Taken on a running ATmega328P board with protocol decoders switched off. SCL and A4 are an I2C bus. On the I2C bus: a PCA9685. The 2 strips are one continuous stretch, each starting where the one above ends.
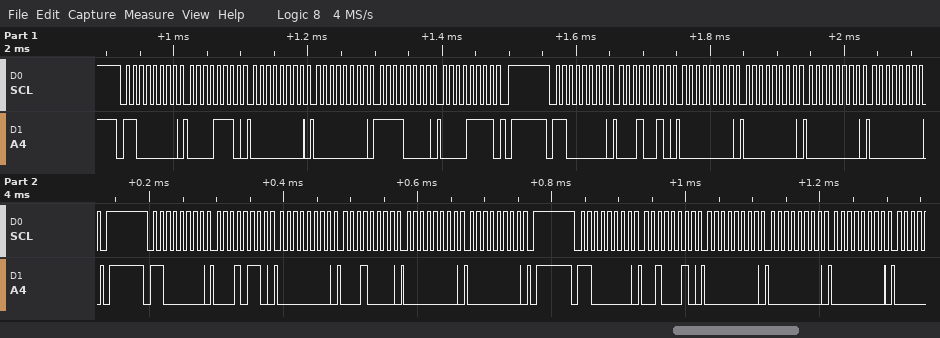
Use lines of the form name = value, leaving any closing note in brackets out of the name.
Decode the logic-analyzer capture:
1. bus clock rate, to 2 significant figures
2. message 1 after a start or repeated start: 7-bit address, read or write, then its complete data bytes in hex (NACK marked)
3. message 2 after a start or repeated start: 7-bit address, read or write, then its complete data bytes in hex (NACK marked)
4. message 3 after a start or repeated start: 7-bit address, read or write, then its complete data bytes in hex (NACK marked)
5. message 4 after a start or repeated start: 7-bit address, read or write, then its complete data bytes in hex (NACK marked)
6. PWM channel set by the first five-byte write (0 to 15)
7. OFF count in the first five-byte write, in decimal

bus clock rate, to 2 significant figures = 100 kHz
message 1 after a start or repeated start: 7-bit address, read or write, then its complete data bytes in hex = 0x60 write: 0E 00 00 F0 0F
message 2 after a start or repeated start: 7-bit address, read or write, then its complete data bytes in hex = 0x60 write: 12 00 00 00 00
message 3 after a start or repeated start: 7-bit address, read or write, then its complete data bytes in hex = 0x60 write: 16 00 10 00 00
message 4 after a start or repeated start: 7-bit address, read or write, then its complete data bytes in hex = 0x60 write: 22 00 00 00
PWM channel set by the first five-byte write = 2
OFF count in the first five-byte write, in decimal = 4080
